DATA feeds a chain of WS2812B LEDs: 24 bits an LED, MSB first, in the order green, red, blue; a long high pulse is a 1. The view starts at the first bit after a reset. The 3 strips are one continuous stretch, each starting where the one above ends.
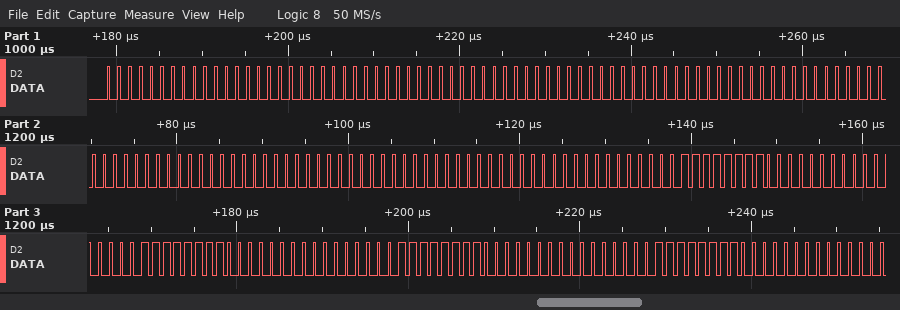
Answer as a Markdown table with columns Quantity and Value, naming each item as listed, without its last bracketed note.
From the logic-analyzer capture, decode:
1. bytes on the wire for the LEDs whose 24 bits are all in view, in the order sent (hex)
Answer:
| Quantity | Value |
|---|---|
| bytes on the wire for the LEDs whose 24 bits are all in view, in the order sent | 00 00 00 00 00 00 00 00 00 00 00 00 00 00 00 00 FF 00 00 FF 00 00 FF 00 00 FF 00 |
